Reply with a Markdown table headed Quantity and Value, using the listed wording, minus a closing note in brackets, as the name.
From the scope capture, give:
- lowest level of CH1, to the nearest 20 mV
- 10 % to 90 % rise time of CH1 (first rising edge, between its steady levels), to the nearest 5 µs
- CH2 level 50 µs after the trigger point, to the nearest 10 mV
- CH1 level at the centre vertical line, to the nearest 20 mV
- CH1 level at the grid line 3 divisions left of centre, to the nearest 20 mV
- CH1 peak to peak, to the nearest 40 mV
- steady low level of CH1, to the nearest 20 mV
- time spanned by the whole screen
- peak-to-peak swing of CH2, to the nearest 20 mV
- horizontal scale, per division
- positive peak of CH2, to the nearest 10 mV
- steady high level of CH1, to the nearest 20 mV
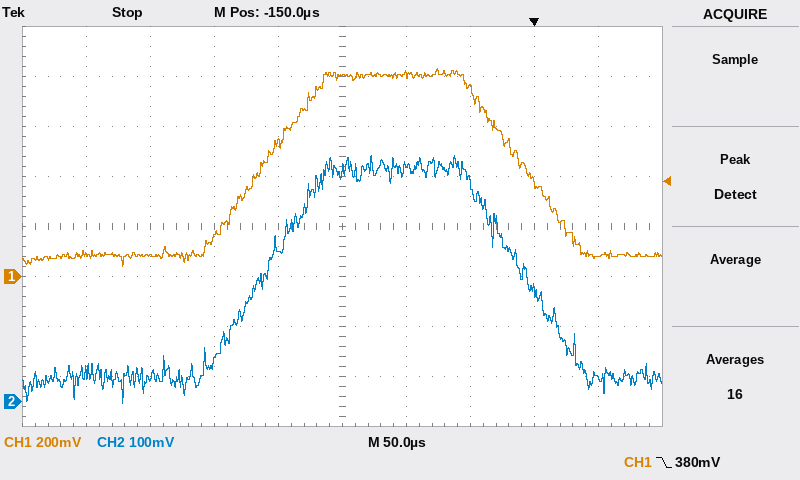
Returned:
| Quantity | Value |
|---|---|
| lowest level of CH1, to the nearest 20 mV | 40 mV |
| 10 % to 90 % rise time of CH1 (first rising edge, between its steady levels), to the nearest 5 µs | 80 µs |
| CH2 level 50 µs after the trigger point, to the nearest 10 mV | 50 mV |
| CH1 level at the centre vertical line, to the nearest 20 mV | 800 mV |
| CH1 level at the grid line 3 divisions left of centre, to the nearest 20 mV | 80 mV |
| CH1 peak to peak, to the nearest 40 mV | 800 mV |
| steady low level of CH1, to the nearest 20 mV | 80 mV |
| time spanned by the whole screen | 500 µs |
| peak-to-peak swing of CH2, to the nearest 20 mV | 500 mV |
| horizontal scale, per division | 50 µs |
| positive peak of CH2, to the nearest 10 mV | 490 mV |
| steady high level of CH1, to the nearest 20 mV | 800 mV |
